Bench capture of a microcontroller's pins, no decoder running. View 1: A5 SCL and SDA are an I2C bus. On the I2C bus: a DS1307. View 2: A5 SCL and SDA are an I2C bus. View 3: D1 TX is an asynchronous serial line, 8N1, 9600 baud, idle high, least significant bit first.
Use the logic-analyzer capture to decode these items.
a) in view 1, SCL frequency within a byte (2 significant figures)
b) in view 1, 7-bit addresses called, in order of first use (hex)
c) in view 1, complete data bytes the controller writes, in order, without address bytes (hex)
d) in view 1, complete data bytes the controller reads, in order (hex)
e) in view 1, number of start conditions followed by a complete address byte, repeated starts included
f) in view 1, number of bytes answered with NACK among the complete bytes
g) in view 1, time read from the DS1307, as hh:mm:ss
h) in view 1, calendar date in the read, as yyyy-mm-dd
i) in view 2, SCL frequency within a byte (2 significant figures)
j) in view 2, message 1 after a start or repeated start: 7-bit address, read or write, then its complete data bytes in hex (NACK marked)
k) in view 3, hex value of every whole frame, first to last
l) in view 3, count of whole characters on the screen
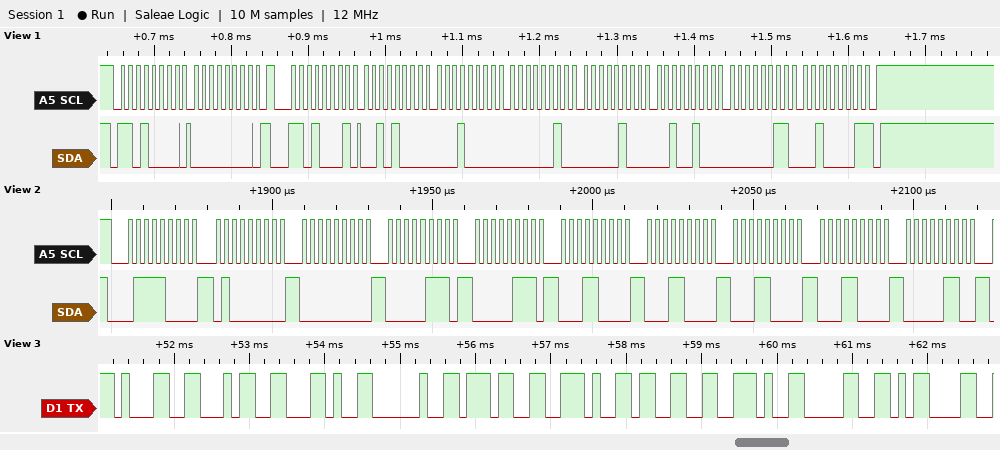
100 kHz
0x68
00
28 10 02 04 24 03 21
2
1
02:10:28
2021-03-24
400 kHz
0x3C write: 40 00 07 07 18 18 18 18 06
31 34 2C 20 37 2E 33 2E 30 0D
10
